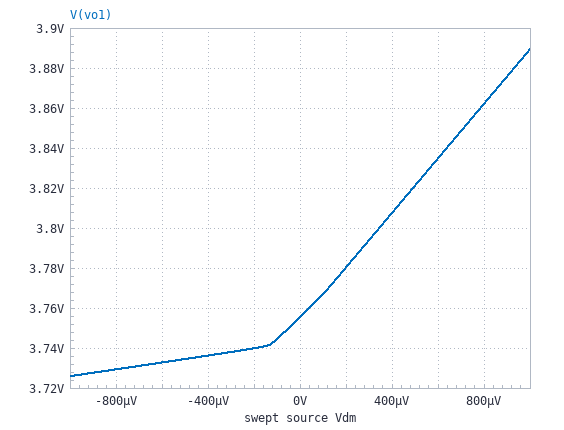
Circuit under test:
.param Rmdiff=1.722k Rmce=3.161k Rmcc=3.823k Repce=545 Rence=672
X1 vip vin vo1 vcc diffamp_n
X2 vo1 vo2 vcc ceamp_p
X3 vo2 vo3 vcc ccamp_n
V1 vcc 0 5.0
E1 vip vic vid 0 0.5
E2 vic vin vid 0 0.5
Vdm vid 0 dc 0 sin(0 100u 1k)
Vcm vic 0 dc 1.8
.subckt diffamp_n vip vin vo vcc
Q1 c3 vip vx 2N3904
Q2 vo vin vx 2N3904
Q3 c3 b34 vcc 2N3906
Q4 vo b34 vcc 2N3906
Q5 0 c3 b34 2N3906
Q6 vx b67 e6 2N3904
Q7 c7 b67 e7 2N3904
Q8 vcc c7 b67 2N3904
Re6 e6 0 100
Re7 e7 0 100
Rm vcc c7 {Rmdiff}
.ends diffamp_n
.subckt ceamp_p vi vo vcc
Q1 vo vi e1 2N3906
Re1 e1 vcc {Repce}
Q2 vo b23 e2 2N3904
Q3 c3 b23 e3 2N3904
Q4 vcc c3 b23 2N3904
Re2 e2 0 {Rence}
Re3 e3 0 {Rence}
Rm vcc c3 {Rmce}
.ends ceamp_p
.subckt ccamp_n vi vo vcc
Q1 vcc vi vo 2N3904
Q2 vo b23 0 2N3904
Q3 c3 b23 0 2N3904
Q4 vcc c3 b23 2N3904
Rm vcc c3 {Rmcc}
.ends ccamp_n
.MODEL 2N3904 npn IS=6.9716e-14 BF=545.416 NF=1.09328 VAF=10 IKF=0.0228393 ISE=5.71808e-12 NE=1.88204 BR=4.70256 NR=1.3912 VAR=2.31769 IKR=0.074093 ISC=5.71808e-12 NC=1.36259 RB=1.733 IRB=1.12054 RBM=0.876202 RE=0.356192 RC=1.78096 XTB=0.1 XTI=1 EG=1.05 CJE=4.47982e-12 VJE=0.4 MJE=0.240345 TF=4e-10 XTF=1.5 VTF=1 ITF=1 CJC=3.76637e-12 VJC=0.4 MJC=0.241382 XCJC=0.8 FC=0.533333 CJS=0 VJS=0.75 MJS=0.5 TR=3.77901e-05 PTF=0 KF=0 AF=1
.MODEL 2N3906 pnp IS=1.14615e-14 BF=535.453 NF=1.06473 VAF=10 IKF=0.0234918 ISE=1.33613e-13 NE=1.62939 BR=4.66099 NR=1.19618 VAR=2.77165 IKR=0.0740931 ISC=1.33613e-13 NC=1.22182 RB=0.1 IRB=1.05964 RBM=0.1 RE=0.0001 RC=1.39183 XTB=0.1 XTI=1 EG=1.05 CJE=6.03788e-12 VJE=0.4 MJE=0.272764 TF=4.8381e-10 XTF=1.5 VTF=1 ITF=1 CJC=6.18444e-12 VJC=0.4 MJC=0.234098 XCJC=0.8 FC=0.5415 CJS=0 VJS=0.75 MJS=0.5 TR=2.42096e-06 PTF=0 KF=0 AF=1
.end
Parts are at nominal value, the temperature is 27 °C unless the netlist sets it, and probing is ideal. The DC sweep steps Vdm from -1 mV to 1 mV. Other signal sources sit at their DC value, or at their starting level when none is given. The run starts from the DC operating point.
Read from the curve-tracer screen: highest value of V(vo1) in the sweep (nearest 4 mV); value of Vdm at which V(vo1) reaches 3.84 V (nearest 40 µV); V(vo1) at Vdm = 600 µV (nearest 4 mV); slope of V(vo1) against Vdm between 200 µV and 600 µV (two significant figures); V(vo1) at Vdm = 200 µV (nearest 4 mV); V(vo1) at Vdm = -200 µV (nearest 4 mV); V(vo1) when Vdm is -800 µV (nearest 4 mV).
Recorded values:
3.888 V
640 µV
3.836 V
140 V/V
3.780 V
3.740 V
3.728 V
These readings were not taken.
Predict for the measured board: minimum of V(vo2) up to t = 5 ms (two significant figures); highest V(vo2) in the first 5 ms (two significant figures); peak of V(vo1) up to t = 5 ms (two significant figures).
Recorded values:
1.0 V
3.8 V
3.8 V
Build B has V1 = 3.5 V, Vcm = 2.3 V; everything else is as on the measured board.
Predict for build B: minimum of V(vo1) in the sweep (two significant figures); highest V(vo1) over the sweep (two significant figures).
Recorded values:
2.4 V
2.5 V
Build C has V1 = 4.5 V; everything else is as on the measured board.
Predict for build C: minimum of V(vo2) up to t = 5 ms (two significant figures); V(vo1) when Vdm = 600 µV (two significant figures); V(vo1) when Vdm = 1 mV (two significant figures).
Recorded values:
3.9 V
3.3 V
3.4 V
